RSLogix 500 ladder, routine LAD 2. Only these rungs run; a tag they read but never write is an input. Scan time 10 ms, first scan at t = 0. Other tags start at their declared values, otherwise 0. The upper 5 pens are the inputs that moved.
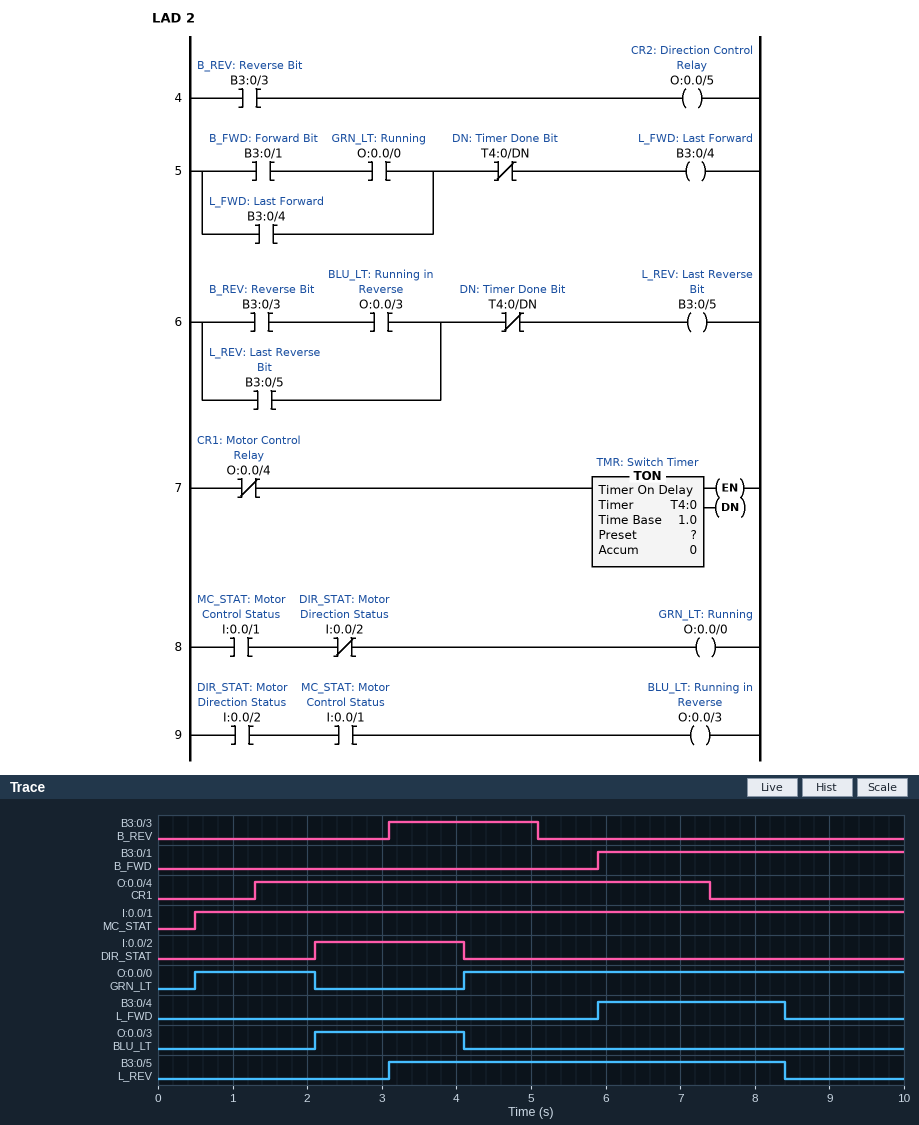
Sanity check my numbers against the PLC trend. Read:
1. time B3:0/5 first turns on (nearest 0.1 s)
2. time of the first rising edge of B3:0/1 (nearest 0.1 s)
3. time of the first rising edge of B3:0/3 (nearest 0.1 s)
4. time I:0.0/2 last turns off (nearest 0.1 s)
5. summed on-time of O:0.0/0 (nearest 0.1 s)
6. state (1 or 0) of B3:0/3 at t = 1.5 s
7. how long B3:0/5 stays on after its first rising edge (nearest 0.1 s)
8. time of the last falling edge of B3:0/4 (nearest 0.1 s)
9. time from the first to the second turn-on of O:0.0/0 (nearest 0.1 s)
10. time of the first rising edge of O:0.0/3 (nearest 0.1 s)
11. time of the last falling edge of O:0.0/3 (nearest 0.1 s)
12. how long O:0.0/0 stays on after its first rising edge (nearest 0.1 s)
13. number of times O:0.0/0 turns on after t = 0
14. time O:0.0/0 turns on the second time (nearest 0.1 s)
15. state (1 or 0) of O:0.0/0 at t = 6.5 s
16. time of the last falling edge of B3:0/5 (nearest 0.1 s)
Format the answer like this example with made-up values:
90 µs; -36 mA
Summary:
3.1 s; 5.9 s; 3.1 s; 4.1 s; 7.5 s; 0; 5.3 s; 8.4 s; 3.6 s; 2.1 s; 4.1 s; 1.6 s; 2; 4.1 s; 1; 8.4 s
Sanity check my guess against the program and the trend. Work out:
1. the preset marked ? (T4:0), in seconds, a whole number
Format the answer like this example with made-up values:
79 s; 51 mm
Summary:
1 s
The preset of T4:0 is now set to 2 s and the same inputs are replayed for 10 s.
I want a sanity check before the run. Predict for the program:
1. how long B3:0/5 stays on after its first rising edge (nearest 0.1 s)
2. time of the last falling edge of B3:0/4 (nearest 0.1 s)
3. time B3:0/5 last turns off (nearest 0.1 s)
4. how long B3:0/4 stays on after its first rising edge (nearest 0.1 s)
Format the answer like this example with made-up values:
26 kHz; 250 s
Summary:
6.3 s; 9.4 s; 9.4 s; 3.5 s
